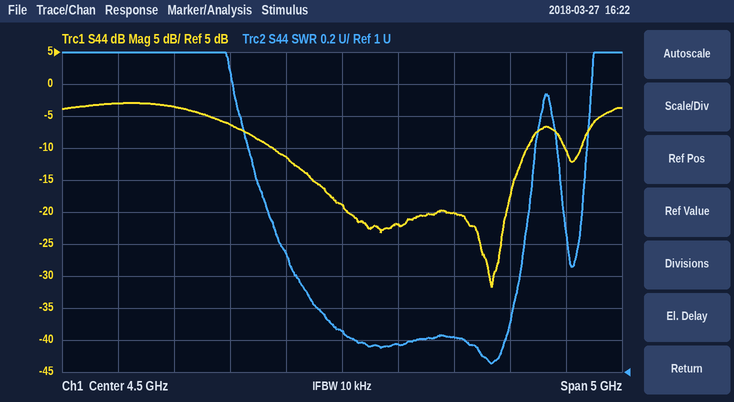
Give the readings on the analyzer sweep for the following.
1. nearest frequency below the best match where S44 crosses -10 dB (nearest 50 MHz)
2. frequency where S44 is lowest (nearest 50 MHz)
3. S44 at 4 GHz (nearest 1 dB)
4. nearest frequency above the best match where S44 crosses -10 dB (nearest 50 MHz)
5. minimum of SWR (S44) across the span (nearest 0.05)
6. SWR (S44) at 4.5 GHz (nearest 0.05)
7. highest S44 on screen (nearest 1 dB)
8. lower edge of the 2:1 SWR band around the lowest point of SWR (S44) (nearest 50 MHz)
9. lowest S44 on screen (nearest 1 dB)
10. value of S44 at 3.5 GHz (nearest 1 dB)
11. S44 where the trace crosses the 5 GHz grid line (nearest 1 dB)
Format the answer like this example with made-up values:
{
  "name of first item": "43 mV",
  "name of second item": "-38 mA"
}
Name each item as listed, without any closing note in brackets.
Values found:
{
  "nearest frequency below the best match where S44 crosses -10 dB": "3.90 GHz",
  "frequency where S44 is lowest": "5.85 GHz",
  "S44 at 4 GHz": "-11 dB",
  "nearest frequency above the best match where S44 crosses -10 dB": "6.15 GHz",
  "minimum of SWR (S44) across the span": "1.05",
  "SWR (S44) at 4.5 GHz": "1.25",
  "highest S44 on screen": "-3 dB",
  "lower edge of the 2:1 SWR band around the lowest point of SWR (S44)": "3.85 GHz",
  "lowest S44 on screen": "-32 dB",
  "value of S44 at 3.5 GHz": "-6 dB",
  "S44 where the trace crosses the 5 GHz grid line": "-22 dB"
}
